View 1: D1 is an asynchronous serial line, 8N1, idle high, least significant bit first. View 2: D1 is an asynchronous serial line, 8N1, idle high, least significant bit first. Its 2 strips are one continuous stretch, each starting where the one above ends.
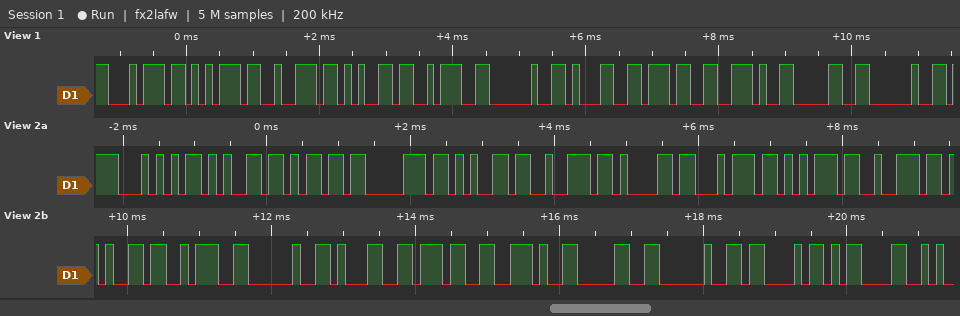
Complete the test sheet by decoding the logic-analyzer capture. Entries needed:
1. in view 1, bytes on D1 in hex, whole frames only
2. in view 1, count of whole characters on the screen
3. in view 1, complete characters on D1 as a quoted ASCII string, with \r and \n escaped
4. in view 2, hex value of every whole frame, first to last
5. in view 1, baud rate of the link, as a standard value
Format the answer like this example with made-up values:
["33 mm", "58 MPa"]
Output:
["74 75 72 65 3A 20 31 37 2E 30 20", "11", "\"ture: 17.0 \"", "0x54 0x65 0x6D 0x70 0x65 0x72 0x61 0x74 0x75 0x72 0x65 0x3A 0x20 0x31 0x37 0x2E 0x30 0x20 0x43 0x0D", "9600 baud"]
